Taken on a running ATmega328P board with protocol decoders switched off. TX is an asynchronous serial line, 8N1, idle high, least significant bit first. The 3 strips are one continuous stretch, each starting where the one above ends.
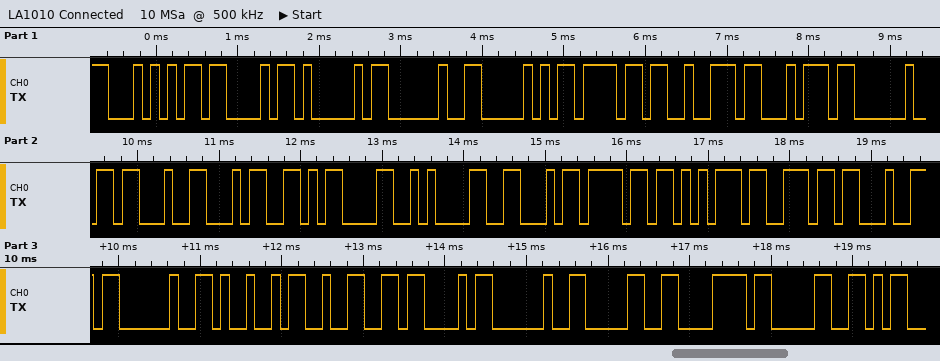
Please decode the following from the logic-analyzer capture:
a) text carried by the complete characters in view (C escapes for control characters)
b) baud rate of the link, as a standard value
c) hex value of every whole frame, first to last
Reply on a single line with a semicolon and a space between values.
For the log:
"TCA Port #4\r\nFound I2C 0x0"; 9600 baud; 54 43 41 20 50 6F 72 74 20 23 34 0D 0A 46 6F 75 6E 64 20 49 32 43 20 30 78 30
